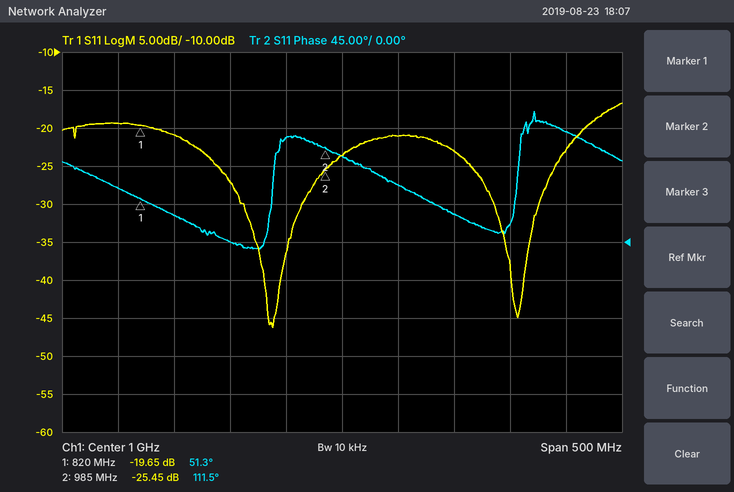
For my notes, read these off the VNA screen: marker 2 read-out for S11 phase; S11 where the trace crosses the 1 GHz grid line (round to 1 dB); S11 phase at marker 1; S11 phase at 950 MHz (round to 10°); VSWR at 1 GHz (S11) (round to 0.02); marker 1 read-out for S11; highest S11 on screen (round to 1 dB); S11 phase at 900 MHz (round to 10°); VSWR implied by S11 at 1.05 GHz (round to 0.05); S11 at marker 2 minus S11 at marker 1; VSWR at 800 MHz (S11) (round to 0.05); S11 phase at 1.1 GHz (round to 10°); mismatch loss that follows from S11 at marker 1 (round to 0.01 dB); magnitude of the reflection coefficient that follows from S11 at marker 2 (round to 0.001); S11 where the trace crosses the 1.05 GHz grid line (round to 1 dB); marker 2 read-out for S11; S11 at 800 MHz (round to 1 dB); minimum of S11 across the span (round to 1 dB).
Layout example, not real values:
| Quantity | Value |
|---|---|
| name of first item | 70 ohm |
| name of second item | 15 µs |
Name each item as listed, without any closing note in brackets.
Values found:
| Quantity | Value |
|---|---|
| marker 2 read-out for S11 phase | 111.5° |
| S11 where the trace crosses the 1 GHz grid line | -24 dB |
| S11 phase at marker 1 | 51.3° |
| S11 phase at 950 MHz | 120° |
| VSWR at 1 GHz (S11) | 1.14 |
| marker 1 read-out for S11 | -19.65 dB |
| highest S11 on screen | -17 dB |
| S11 phase at 900 MHz | 0° |
| VSWR implied by S11 at 1.05 GHz | 1.20 |
| S11 at marker 2 minus S11 at marker 1 | -5.80 dB |
| VSWR at 800 MHz (S11) | 1.25 |
| S11 phase at 1.1 GHz | 30° |
| mismatch loss that follows from S11 at marker 1 | 0.05 dB |
| magnitude of the reflection coefficient that follows from S11 at marker 2 | 0.053 |
| S11 where the trace crosses the 1.05 GHz grid line | -21 dB |
| marker 2 read-out for S11 | -25.45 dB |
| S11 at 800 MHz | -19 dB |
| minimum of S11 across the span | -46 dB |
